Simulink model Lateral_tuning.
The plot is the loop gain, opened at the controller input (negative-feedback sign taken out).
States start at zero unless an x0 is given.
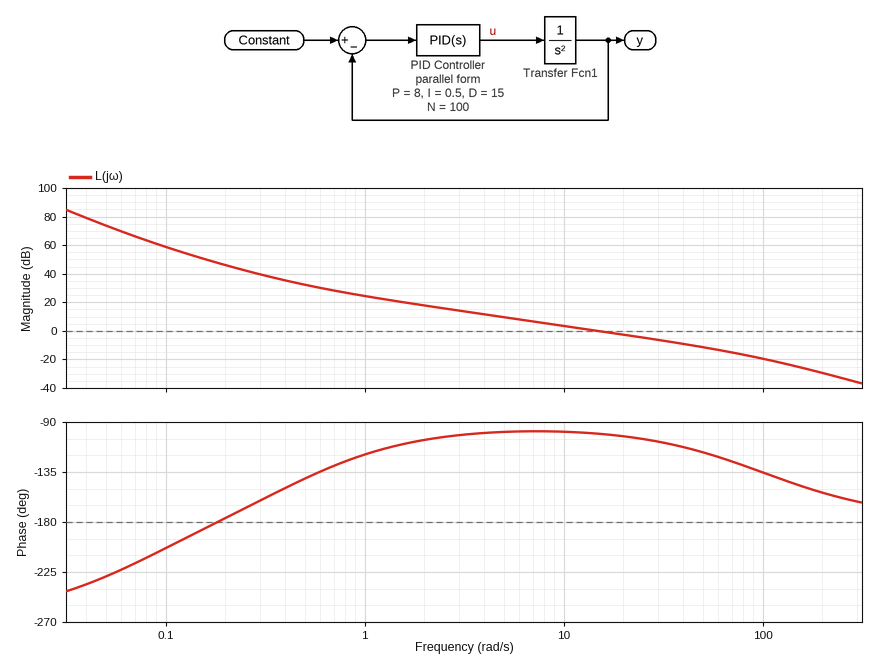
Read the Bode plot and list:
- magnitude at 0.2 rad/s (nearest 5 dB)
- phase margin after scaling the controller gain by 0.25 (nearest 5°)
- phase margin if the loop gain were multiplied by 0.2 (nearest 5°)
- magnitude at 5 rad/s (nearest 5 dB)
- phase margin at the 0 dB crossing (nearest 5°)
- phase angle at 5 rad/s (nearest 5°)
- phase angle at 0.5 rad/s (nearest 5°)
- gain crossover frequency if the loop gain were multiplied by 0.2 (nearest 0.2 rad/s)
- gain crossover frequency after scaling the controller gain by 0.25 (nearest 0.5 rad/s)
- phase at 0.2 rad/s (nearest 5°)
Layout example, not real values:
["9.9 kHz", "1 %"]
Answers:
["45 dB", "80°", "80°", "10 dB", "80°", "-100°", "-140°", "3.0 rad/s", "4.0 rad/s", "-175°"]
